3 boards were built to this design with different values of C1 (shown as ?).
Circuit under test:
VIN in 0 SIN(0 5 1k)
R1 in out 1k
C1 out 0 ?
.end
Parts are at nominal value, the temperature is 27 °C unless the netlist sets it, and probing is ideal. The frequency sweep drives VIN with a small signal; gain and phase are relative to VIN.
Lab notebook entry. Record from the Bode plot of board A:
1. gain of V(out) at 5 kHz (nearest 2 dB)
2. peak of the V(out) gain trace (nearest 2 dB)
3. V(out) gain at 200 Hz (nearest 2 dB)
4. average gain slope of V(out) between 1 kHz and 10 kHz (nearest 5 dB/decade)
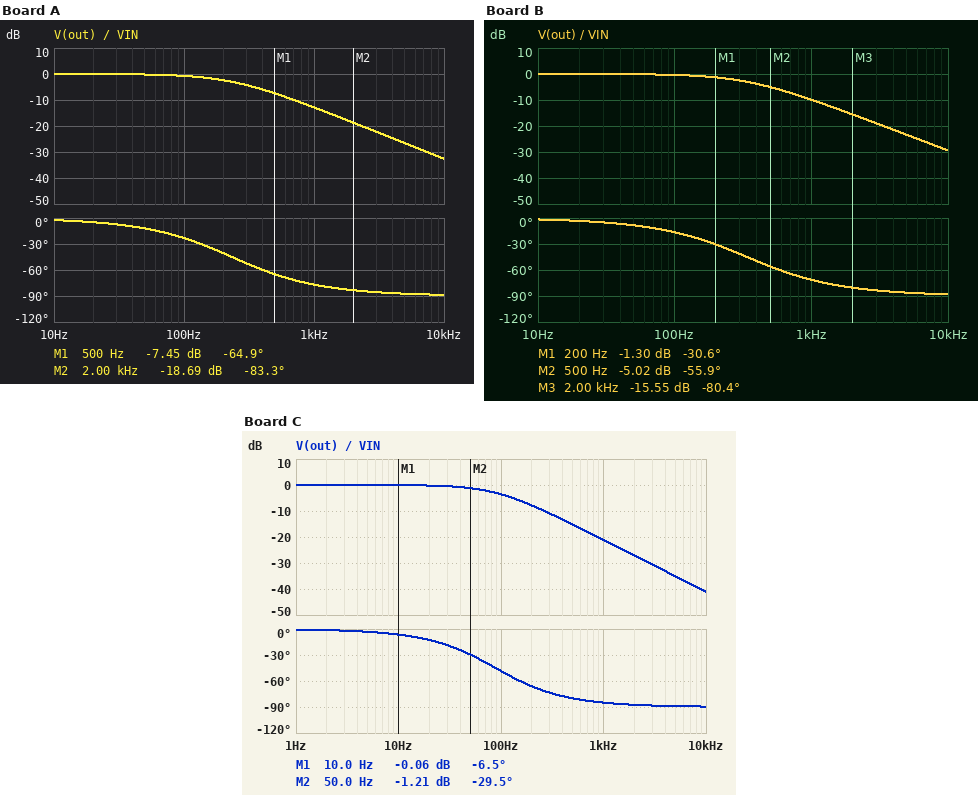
-26 dB
0 dB
-2 dB
-20 dB/decade
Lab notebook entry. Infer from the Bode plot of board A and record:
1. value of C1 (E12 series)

680 nF
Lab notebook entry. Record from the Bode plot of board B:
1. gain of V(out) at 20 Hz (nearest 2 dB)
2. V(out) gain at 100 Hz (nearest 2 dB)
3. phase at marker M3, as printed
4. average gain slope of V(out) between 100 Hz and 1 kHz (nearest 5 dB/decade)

0 dB
0 dB
-80.4 deg
-10 dB/decade
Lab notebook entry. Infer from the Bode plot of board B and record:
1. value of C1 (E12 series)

470 nF
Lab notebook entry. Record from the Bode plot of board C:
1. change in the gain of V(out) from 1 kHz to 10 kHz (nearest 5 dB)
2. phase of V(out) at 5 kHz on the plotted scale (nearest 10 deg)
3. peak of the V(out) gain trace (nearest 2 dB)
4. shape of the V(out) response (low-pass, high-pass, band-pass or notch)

-20 dB
-90 deg
0 dB
low-pass
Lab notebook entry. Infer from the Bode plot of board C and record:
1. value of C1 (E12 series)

1.8 µF
